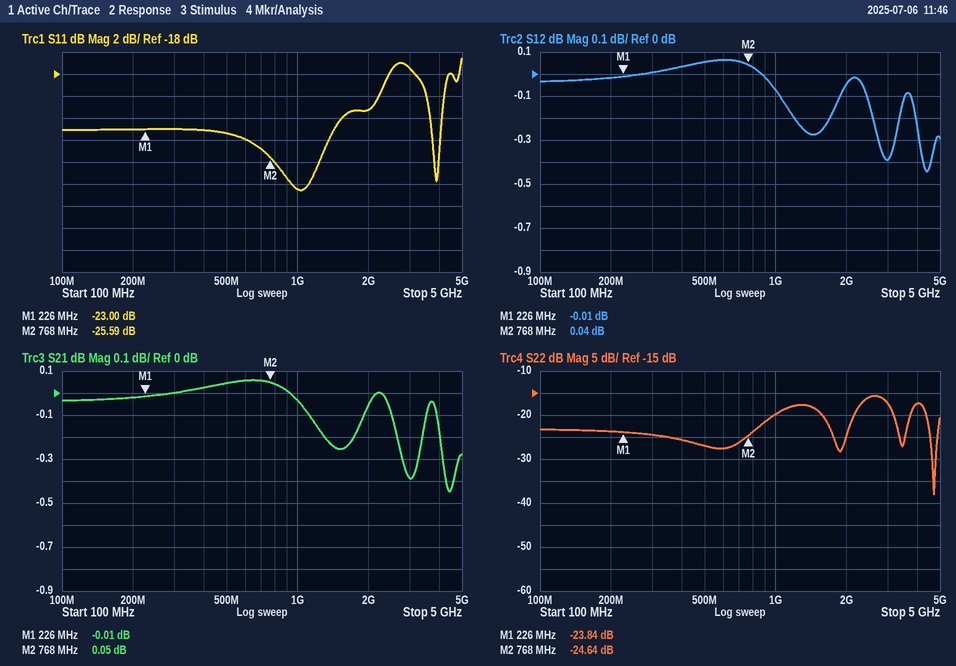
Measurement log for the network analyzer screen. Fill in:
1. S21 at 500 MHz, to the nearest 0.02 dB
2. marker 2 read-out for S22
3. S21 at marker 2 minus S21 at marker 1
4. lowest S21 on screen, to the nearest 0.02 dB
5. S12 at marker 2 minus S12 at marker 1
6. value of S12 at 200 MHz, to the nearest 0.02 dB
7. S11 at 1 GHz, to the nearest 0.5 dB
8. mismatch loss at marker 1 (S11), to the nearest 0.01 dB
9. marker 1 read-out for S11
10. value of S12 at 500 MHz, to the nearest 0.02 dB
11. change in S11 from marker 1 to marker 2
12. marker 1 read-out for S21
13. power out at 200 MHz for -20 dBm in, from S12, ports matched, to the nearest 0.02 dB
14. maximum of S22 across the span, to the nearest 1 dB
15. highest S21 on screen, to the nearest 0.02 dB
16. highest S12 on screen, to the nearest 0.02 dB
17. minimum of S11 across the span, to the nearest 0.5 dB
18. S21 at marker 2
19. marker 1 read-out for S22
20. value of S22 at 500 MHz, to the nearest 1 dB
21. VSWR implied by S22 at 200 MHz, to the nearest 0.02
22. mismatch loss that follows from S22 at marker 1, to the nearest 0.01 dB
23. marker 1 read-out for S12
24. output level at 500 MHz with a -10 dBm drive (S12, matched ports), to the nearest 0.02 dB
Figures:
0.04 dB
-24.64 dB
0.06 dB
-0.44 dB
0.05 dB
-0.02 dB
-28.5 dB
0.02 dB
-23.00 dB
0.06 dB
-2.59 dB
-0.01 dB
-20.02 dBm
-16 dB
0.06 dB
0.06 dB
-28.5 dB
0.05 dB
-23.84 dB
-27 dB
1.14
0.02 dB
-0.01 dB
-9.94 dBm
